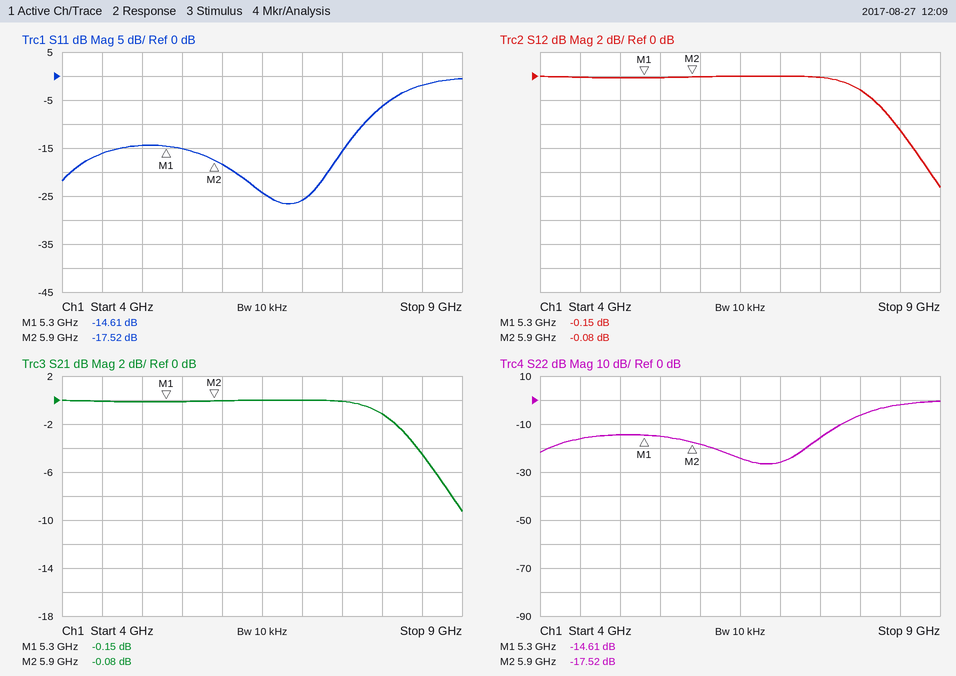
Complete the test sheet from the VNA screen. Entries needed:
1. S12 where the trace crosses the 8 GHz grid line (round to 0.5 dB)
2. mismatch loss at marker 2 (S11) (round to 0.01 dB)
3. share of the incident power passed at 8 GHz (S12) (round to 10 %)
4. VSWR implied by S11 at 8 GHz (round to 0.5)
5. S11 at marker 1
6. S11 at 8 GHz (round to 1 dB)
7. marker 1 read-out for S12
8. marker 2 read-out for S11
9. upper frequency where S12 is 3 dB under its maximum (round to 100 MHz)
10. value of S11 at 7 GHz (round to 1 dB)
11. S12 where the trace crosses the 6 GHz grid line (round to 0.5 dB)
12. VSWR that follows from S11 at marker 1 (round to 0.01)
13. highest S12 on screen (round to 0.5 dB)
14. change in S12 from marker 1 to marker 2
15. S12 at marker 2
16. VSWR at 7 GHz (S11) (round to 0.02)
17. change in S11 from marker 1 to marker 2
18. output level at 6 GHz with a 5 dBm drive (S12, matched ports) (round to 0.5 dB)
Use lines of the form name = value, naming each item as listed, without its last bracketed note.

S12 where the trace crosses the 8 GHz grid line = -1.0 dB
mismatch loss at marker 2 (S11) = 0.08 dB
share of the incident power passed at 8 GHz (S12) = 80 %
VSWR implied by S11 at 8 GHz = 3.0
S11 at marker 1 = -14.61 dB
S11 at 8 GHz = -6 dB
marker 1 read-out for S12 = -0.15 dB
marker 2 read-out for S11 = -17.52 dB
upper frequency where S12 is 3 dB under its maximum = 8.3 GHz
value of S11 at 7 GHz = -26 dB
S12 where the trace crosses the 6 GHz grid line = 0.0 dB
VSWR that follows from S11 at marker 1 = 1.46
highest S12 on screen = 0.0 dB
change in S12 from marker 1 to marker 2 = 0.07 dB
S12 at marker 2 = -0.08 dB
VSWR at 7 GHz (S11) = 1.10
change in S11 from marker 1 to marker 2 = -2.91 dB
output level at 6 GHz with a 5 dBm drive (S12, matched ports) = 5.0 dBm
